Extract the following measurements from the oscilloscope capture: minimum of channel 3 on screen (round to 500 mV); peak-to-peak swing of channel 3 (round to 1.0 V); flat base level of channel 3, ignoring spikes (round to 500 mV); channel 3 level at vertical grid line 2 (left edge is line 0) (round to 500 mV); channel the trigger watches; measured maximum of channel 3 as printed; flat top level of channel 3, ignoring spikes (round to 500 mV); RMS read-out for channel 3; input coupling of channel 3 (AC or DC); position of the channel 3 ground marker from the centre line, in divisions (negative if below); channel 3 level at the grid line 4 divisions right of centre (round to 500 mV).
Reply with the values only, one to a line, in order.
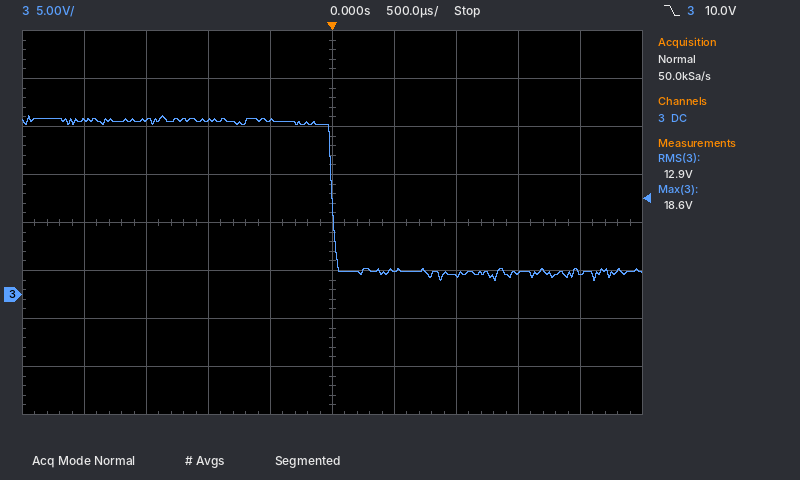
1.5 V
17.0 V
2.5 V
18.0 V
channel 3
18.6 V
18.0 V
12.9 V
DC
-1.5 div
2.5 V
